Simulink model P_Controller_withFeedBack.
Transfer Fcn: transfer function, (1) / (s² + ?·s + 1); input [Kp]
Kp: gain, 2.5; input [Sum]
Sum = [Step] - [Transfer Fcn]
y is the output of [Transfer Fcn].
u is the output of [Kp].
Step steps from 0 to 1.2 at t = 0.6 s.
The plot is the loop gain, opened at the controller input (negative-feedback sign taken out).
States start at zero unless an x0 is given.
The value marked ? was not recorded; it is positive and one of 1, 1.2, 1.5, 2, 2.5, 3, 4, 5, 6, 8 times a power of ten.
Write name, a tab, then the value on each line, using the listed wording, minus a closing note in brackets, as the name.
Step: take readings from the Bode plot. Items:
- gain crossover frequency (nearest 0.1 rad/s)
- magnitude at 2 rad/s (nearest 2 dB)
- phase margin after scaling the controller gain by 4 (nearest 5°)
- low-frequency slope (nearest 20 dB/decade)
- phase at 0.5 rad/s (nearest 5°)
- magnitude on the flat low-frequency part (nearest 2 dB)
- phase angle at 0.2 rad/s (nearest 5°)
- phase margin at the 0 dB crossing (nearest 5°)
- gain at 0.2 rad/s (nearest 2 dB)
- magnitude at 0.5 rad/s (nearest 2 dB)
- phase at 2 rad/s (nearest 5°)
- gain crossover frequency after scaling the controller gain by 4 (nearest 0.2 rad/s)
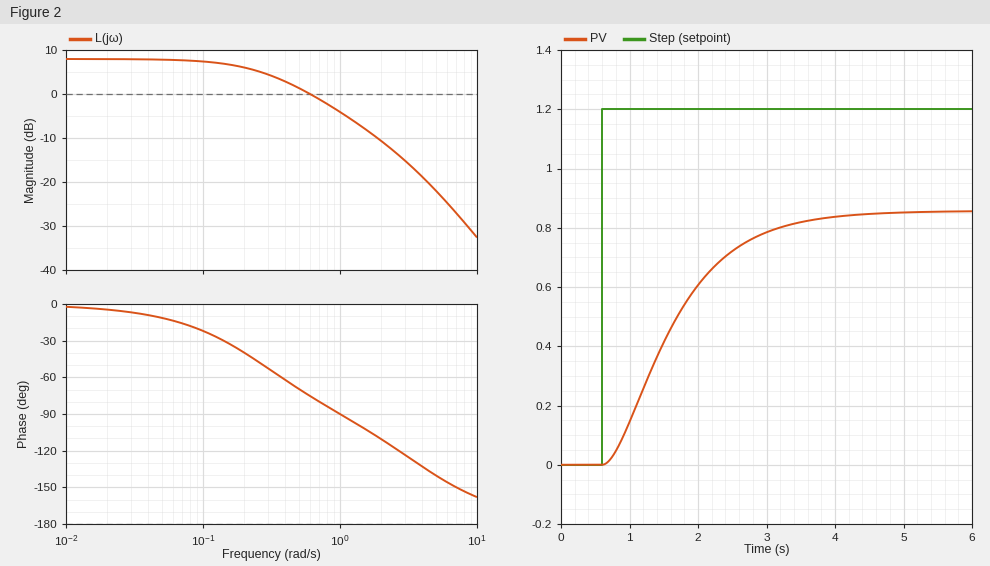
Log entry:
gain crossover frequency	0.6 rad/s
magnitude at 2 rad/s	-10 dB
phase margin after scaling the controller gain by 4	65°
low-frequency slope	0 dB/decade
phase at 0.5 rad/s	-70°
magnitude on the flat low-frequency part	8 dB
phase angle at 0.2 rad/s	-40°
phase margin at the 0 dB crossing	105°
gain at 0.2 rad/s	6 dB
magnitude at 0.5 rad/s	2 dB
phase at 2 rad/s	-110°
gain crossover frequency after scaling the controller gain by 4	2.2 rad/s
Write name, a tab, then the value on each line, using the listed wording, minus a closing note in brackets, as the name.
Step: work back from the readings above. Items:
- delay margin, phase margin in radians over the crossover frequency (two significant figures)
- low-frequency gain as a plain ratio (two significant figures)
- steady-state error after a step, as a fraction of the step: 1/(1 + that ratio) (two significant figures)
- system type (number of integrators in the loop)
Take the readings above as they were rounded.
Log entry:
delay margin, phase margin in radians over the crossover frequency	3.1 s
low-frequency gain as a plain ratio	2.5
steady-state error after a step, as a fraction of the step: 1/(1 + that ratio)	0.29
system type	0
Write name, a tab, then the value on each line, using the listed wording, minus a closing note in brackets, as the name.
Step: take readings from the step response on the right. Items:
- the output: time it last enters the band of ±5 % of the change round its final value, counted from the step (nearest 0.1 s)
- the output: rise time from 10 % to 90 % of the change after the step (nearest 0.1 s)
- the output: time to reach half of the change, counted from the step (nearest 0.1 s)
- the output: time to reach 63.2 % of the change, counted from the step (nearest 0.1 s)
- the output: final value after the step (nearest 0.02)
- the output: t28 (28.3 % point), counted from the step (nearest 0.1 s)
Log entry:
the output: time it last enters the band of ±5 % of the change round its final value, counted from the step	2.8 s
the output: rise time from 10 % to 90 % of the change after the step	2.0 s
the output: time to reach half of the change, counted from the step	0.9 s
the output: time to reach 63.2 % of the change, counted from the step	1.2 s
the output: final value after the step	0.86
the output: t28 (28.3 % point), counted from the step	0.6 s
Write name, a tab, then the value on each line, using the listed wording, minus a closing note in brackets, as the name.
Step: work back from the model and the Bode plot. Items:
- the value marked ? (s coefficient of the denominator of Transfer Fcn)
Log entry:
the value marked ?	4
